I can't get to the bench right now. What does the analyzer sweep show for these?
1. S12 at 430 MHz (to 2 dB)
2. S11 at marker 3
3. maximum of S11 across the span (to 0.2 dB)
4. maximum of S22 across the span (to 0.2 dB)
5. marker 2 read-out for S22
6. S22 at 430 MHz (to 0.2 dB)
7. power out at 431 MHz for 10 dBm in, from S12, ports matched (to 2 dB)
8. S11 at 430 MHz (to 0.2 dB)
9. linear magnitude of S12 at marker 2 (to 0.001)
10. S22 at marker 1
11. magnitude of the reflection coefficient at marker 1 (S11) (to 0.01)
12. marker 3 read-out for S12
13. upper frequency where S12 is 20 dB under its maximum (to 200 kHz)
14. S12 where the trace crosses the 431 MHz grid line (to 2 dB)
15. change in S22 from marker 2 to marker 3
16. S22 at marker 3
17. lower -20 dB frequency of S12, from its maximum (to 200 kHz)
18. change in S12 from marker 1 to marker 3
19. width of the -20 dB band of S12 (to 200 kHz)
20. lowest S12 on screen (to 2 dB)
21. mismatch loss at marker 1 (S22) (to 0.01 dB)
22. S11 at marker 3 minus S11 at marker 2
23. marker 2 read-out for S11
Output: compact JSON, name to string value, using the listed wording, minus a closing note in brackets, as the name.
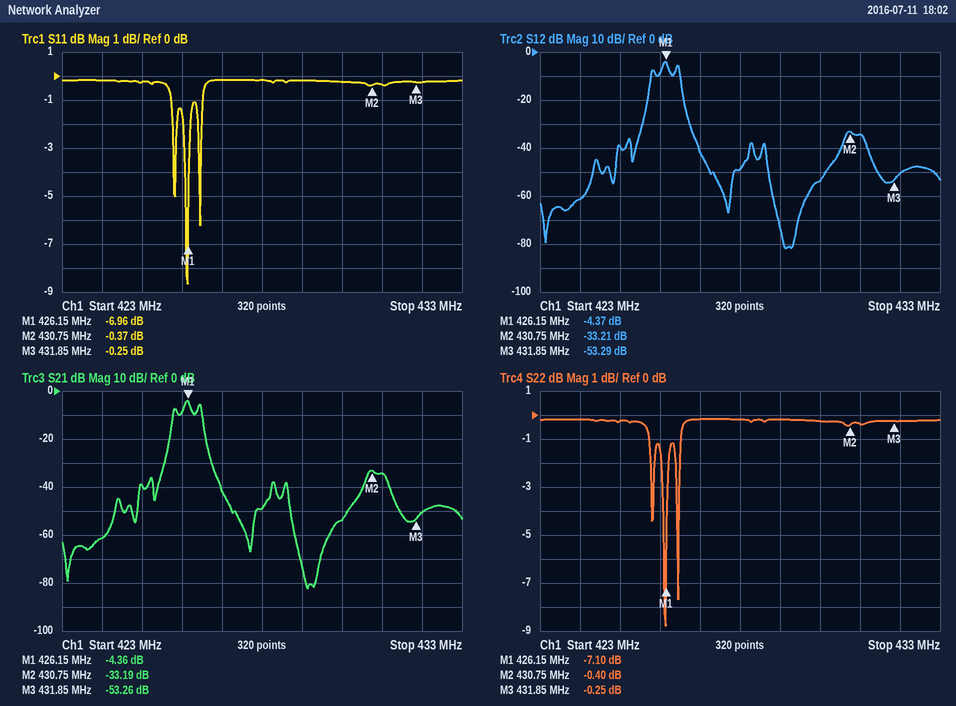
{"S12 at 430 MHz": "-54 dB", "S11 at marker 3": "-0.25 dB", "maximum of S11 across the span": "-0.2 dB", "maximum of S22 across the span": "-0.2 dB", "marker 2 read-out for S22": "-0.40 dB", "S22 at 430 MHz": "-0.2 dB", "power out at 431 MHz for 10 dBm in, from S12, ports matched": "-24 dBm", "S11 at 430 MHz": "-0.2 dB", "linear magnitude of S12 at marker 2": "0.022", "S22 at marker 1": "-7.10 dB", "magnitude of the reflection coefficient at marker 1 (S11)": "0.45", "marker 3 read-out for S12": "-53.29 dB", "upper frequency where S12 is 20 dB under its maximum": "426.6 MHz", "S12 where the trace crosses the 431 MHz grid line": "-34 dB", "change in S22 from marker 2 to marker 3": "0.15 dB", "S22 at marker 3": "-0.25 dB", "lower -20 dB frequency of S12, from its maximum": "425.6 MHz", "change in S12 from marker 1 to marker 3": "-48.92 dB", "width of the -20 dB band of S12": "1.0 MHz", "lowest S12 on screen": "-82 dB", "mismatch loss at marker 1 (S22)": "0.94 dB", "S11 at marker 3 minus S11 at marker 2": "0.12 dB", "marker 2 read-out for S11": "-0.37 dB"}
